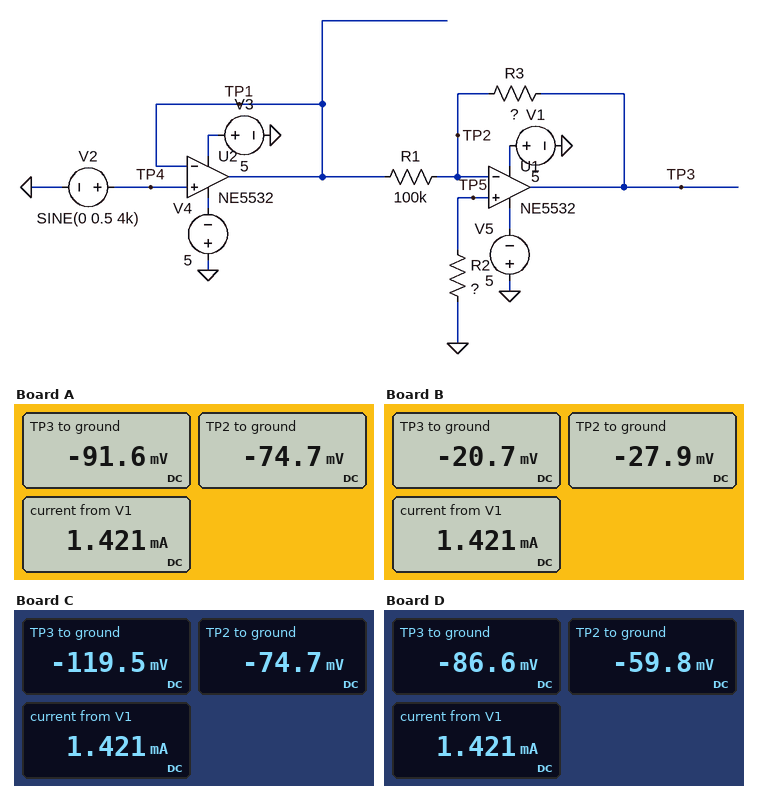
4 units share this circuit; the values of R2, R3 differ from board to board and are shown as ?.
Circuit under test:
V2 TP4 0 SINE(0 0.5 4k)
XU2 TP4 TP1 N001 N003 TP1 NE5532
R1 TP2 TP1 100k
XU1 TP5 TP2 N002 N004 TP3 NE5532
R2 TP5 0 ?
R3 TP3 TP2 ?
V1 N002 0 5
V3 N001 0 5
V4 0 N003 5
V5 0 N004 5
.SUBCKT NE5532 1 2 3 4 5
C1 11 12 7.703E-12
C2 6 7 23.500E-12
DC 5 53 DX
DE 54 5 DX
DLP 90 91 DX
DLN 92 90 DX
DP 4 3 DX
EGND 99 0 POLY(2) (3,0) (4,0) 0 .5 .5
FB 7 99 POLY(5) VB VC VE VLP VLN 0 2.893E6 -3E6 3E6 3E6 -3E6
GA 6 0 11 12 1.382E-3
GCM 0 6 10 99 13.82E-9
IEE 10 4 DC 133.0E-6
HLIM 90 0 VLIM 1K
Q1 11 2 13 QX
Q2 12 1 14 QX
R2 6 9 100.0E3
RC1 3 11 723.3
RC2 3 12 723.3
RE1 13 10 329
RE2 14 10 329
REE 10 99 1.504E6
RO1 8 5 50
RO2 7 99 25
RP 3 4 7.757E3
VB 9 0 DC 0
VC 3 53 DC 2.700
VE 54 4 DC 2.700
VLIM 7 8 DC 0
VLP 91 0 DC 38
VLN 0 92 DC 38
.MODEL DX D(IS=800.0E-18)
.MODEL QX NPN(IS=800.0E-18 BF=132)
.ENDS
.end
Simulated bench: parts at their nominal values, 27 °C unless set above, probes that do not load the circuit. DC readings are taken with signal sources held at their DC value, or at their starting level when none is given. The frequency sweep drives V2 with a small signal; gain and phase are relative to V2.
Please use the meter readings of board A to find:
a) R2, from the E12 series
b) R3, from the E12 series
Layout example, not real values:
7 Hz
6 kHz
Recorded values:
150 kΩ
68 kΩ
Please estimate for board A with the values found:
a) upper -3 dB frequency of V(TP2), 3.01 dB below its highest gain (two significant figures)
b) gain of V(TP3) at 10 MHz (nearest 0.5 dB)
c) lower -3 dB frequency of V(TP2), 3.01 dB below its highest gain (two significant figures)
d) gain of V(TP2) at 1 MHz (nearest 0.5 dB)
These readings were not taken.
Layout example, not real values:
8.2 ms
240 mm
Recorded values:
13 MHz
-16.0 dB
2.8 MHz
-18.0 dB
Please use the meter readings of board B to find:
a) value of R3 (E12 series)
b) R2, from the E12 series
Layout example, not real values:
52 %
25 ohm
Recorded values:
33 kΩ
56 kΩ
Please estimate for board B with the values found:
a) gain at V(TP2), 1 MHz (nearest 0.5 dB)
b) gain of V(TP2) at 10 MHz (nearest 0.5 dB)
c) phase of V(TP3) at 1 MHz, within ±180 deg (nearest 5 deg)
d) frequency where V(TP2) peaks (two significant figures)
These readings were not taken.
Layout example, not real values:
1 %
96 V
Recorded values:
-27.0 dB
-12.0 dB
160 deg
8.2 MHz
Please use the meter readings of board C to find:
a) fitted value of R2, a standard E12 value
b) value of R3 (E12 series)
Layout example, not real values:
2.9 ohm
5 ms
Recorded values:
150 kΩ
180 kΩ
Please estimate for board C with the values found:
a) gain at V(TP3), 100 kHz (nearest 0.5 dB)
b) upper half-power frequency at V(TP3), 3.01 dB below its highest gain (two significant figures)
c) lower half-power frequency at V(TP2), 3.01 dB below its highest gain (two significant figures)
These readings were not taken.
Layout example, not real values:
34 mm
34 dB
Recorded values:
5.0 dB
1.8 MHz
1.7 MHz
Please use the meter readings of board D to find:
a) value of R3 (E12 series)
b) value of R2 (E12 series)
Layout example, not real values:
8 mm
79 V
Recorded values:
270 kΩ
120 kΩ
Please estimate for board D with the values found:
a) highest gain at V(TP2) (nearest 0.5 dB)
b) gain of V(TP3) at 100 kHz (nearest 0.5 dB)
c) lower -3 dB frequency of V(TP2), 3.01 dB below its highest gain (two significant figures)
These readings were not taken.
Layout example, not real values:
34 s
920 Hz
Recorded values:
-4.0 dB
8.5 dB
1.3 MHz
